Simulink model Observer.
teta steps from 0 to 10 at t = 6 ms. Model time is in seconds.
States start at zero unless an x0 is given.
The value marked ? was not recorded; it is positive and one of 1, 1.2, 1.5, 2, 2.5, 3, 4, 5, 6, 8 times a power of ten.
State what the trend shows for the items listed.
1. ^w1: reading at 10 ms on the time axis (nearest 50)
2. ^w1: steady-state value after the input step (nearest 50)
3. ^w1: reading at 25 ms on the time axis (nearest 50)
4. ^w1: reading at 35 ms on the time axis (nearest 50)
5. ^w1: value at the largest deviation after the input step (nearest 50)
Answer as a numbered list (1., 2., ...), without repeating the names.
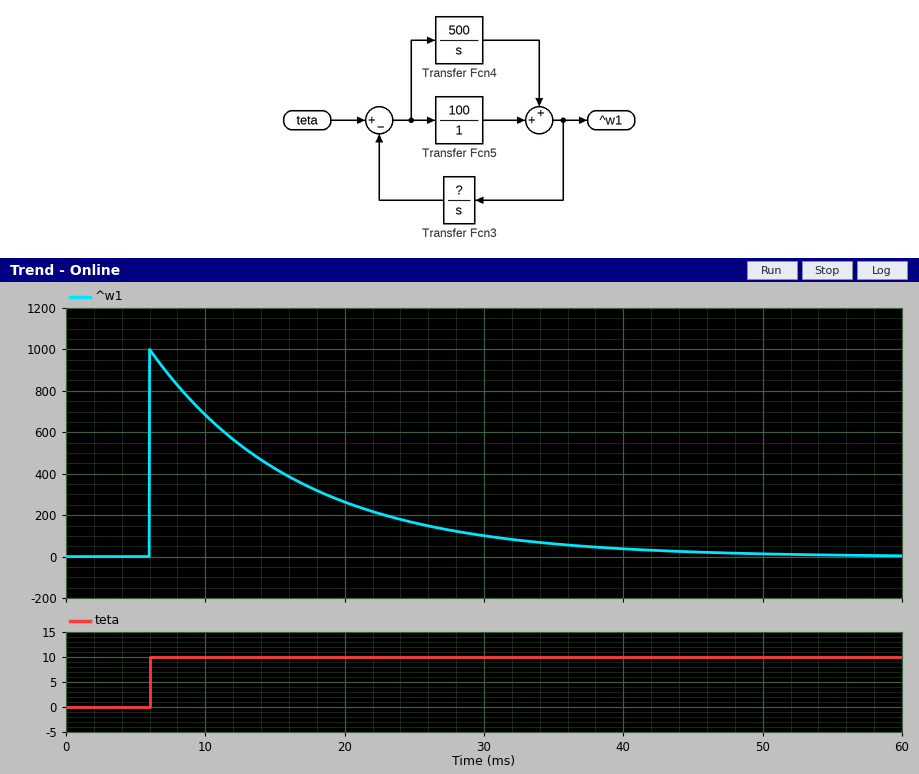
1. 700
2. 0
3. 150
4. 50
5. 1000
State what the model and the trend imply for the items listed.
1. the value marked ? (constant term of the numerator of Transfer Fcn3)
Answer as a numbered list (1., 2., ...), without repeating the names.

1. 1
